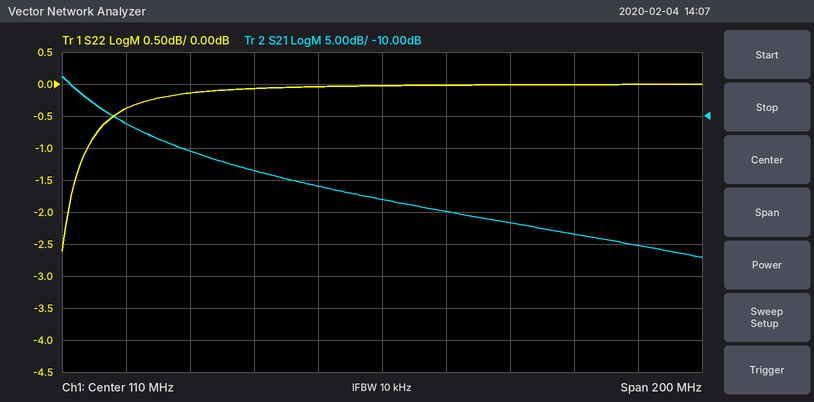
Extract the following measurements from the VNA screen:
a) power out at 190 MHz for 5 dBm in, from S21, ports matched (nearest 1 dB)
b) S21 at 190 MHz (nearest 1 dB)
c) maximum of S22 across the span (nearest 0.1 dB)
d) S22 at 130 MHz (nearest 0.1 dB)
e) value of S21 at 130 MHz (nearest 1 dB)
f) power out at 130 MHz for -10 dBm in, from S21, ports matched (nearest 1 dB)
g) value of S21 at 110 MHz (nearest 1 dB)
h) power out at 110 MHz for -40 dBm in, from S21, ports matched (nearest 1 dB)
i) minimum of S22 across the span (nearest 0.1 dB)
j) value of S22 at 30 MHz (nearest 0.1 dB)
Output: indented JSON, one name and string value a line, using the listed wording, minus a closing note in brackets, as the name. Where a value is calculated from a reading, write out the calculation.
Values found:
{
  "power out at 190 MHz for 5 dBm in, from S21, ports matched": "5 dBm + (-30 dB) = -25 dBm",
  "S21 at 190 MHz": "-30 dB",
  "maximum of S22 across the span": "0.0 dB",
  "S22 at 130 MHz": "0.0 dB",
  "value of S21 at 130 MHz": "-25 dB",
  "power out at 130 MHz for -10 dBm in, from S21, ports matched": "-10 dBm + (-25 dB) = -35 dBm",
  "value of S21 at 110 MHz": "-23 dB",
  "power out at 110 MHz for -40 dBm in, from S21, ports matched": "-40 dBm + (-23 dB) = -63 dBm",
  "minimum of S22 across the span": "-2.6 dB",
  "value of S22 at 30 MHz": "-0.4 dB"
}
